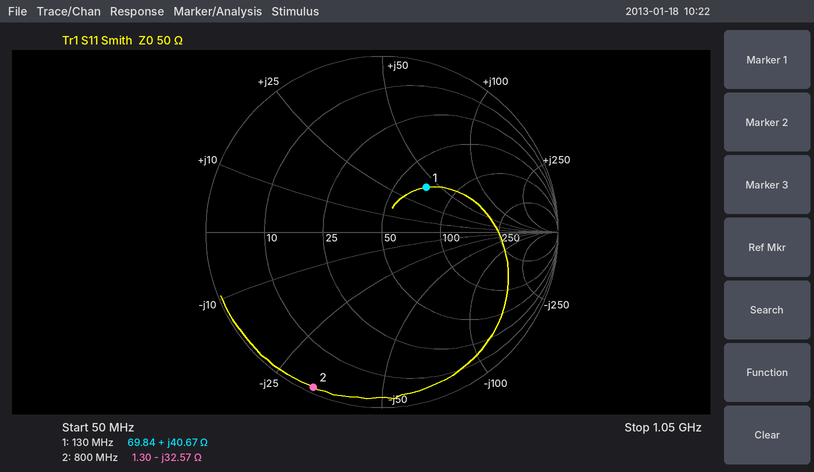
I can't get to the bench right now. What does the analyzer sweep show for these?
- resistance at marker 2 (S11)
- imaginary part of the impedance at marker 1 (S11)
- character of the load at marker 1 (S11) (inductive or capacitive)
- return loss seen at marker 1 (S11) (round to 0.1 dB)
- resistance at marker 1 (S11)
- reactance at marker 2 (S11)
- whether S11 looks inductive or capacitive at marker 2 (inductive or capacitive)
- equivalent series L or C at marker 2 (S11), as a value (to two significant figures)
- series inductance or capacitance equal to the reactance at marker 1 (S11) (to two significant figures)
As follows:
1.30 Ω
+40.67 Ω
inductive
8.9 dB
69.84 Ω
-32.57 Ω
capacitive
6.1 pF
50 nH
